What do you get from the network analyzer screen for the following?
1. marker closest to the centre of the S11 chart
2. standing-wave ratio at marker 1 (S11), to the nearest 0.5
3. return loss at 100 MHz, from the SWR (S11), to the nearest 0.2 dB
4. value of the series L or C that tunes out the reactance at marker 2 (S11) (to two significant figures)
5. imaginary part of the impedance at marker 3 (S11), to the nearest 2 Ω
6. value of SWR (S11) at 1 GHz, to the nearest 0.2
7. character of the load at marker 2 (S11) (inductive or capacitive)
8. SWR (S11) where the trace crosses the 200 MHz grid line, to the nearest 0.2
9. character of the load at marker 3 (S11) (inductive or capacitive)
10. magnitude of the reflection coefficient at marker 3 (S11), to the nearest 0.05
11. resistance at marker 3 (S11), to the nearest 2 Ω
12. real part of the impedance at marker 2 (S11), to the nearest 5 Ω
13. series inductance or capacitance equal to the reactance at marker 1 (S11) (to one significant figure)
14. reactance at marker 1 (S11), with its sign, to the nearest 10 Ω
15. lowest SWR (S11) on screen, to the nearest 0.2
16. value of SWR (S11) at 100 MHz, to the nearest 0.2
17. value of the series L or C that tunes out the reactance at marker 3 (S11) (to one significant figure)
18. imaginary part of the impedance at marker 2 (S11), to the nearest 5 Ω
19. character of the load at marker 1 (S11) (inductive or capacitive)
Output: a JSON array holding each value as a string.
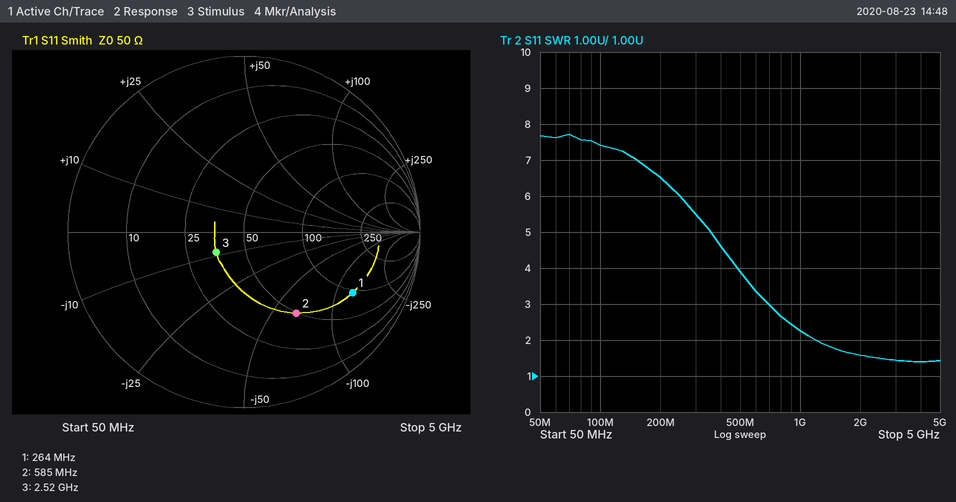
["marker 3", "6.0", "2.4 dB", "18 nH", "-8 Ω", "2.2", "capacitive", "6.6", "capacitive", "0.20", "36 Ω", "50 Ω", "5 pF", "-130 Ω", "1.4", "7.4", "500 pH", "-65 Ω", "capacitive"]
